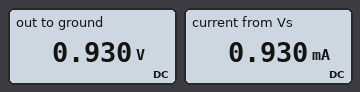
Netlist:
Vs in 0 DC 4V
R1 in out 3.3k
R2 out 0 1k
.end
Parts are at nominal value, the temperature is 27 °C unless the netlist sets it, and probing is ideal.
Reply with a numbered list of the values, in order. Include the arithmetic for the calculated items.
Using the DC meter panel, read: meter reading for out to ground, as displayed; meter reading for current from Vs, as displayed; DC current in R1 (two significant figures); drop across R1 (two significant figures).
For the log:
1. 0.930 V
2. 0.930 mA
3. (4 V - 930 mV) / 3.3 kΩ = 930 µA
4. 4 V - 930 mV = 3.1 V
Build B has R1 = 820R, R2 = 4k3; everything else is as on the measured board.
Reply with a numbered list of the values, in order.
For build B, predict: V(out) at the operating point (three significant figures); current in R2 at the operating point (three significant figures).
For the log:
1. 3.36 V
2. 781 µA
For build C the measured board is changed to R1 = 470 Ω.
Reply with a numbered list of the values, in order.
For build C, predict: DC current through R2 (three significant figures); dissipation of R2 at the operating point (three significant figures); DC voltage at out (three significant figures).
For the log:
1. 2.72 mA
2. 7.40 mW
3. 2.72 V
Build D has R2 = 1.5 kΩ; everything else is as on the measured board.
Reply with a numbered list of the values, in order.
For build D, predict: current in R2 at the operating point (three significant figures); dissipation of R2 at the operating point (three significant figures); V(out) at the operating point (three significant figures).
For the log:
1. 833 µA
2. 1.04 mW
3. 1.25 V
